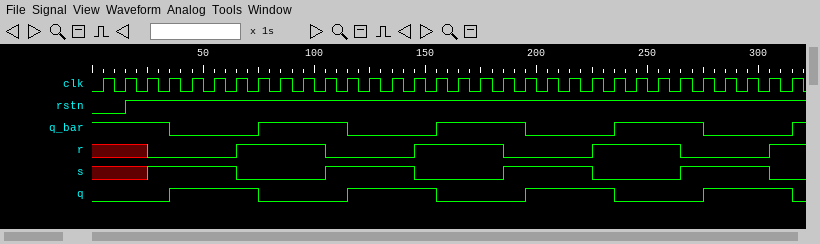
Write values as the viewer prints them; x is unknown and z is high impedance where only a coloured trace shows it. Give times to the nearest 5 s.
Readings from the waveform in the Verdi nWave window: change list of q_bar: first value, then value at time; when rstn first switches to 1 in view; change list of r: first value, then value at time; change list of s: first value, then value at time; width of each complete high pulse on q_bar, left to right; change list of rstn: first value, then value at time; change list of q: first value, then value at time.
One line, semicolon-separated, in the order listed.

1, 0 at 35 s, 1 at 75 s, 0 at 115 s, 1 at 155 s, 0 at 195 s, 1 at 235 s, 0 at 275 s, 1 at 315 s; 15 s; x, 0 at 25 s, 1 at 65 s, 0 at 105 s, 1 at 145 s, 0 at 185 s, 1 at 225 s, 0 at 265 s, 1 at 305 s; x, 1 at 25 s, 0 at 65 s, 1 at 105 s, 0 at 145 s, 1 at 185 s, 0 at 225 s, 1 at 265 s, 0 at 305 s; 40 s, 40 s, 40 s; 0, 1 at 15 s; 0, 1 at 35 s, 0 at 75 s, 1 at 115 s, 0 at 155 s, 1 at 195 s, 0 at 235 s, 1 at 275 s, 0 at 315 s
